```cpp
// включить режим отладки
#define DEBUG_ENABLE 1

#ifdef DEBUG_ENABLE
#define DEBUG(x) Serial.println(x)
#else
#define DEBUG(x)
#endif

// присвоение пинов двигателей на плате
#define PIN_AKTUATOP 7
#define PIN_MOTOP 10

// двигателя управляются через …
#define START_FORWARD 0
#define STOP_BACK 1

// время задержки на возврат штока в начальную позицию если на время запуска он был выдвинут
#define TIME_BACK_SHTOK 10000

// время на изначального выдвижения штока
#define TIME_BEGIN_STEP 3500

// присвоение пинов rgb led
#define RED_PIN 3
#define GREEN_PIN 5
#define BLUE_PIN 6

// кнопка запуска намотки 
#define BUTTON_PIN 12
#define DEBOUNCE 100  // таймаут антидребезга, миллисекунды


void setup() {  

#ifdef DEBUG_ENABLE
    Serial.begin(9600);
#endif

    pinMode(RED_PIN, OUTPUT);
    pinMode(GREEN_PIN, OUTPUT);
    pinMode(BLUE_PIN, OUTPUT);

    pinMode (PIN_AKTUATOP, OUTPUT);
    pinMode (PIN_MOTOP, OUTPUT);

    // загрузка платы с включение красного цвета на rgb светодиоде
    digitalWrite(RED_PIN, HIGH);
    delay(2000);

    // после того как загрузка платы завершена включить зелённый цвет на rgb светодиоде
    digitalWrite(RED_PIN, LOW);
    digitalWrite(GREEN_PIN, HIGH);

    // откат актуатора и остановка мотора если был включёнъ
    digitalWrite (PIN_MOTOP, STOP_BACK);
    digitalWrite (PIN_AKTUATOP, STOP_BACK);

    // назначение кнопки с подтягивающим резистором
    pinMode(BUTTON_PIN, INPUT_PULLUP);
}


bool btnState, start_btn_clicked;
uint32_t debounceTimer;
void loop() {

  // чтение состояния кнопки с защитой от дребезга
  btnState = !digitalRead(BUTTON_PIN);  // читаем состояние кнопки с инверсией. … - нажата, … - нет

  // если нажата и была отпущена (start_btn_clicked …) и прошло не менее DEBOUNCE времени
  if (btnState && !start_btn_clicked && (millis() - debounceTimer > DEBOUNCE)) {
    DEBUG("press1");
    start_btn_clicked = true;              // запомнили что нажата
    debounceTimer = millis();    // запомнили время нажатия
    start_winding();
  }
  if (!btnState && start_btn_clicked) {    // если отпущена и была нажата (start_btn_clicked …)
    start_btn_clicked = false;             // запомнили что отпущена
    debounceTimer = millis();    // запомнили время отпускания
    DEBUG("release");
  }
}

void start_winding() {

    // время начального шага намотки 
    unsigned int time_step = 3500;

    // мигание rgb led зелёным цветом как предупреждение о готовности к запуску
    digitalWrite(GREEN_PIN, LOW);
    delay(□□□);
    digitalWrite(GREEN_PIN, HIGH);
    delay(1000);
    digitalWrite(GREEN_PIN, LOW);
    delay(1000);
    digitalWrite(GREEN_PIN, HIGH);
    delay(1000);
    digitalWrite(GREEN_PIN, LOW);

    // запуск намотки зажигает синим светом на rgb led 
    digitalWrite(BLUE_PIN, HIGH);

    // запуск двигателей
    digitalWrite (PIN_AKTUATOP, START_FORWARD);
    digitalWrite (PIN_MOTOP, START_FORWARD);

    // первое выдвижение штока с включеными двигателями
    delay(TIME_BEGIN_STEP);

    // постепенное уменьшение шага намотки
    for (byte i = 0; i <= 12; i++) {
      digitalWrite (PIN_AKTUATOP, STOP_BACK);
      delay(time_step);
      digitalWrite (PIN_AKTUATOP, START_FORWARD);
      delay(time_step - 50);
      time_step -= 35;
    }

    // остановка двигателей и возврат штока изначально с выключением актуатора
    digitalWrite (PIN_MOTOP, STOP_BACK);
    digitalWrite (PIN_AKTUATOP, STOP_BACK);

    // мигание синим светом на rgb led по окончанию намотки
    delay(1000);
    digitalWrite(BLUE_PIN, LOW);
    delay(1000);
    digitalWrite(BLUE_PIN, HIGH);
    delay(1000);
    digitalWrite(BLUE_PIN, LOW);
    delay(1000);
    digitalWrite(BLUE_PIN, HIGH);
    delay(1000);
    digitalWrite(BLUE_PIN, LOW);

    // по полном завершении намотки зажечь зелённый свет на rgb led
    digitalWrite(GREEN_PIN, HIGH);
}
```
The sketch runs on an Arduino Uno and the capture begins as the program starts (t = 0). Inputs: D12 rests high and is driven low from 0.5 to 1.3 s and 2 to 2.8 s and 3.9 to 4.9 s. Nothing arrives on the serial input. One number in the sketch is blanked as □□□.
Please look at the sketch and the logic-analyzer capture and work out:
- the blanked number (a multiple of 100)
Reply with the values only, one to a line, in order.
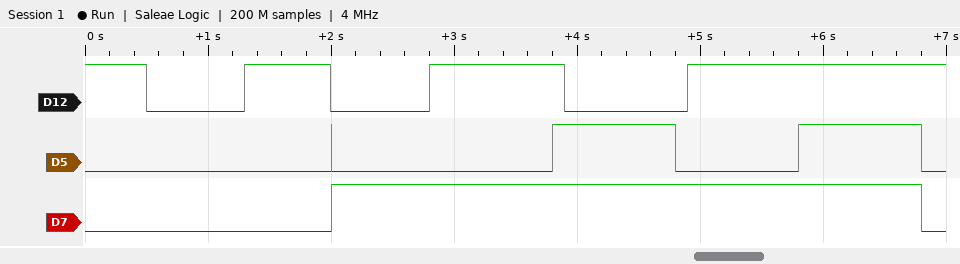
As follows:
1800
